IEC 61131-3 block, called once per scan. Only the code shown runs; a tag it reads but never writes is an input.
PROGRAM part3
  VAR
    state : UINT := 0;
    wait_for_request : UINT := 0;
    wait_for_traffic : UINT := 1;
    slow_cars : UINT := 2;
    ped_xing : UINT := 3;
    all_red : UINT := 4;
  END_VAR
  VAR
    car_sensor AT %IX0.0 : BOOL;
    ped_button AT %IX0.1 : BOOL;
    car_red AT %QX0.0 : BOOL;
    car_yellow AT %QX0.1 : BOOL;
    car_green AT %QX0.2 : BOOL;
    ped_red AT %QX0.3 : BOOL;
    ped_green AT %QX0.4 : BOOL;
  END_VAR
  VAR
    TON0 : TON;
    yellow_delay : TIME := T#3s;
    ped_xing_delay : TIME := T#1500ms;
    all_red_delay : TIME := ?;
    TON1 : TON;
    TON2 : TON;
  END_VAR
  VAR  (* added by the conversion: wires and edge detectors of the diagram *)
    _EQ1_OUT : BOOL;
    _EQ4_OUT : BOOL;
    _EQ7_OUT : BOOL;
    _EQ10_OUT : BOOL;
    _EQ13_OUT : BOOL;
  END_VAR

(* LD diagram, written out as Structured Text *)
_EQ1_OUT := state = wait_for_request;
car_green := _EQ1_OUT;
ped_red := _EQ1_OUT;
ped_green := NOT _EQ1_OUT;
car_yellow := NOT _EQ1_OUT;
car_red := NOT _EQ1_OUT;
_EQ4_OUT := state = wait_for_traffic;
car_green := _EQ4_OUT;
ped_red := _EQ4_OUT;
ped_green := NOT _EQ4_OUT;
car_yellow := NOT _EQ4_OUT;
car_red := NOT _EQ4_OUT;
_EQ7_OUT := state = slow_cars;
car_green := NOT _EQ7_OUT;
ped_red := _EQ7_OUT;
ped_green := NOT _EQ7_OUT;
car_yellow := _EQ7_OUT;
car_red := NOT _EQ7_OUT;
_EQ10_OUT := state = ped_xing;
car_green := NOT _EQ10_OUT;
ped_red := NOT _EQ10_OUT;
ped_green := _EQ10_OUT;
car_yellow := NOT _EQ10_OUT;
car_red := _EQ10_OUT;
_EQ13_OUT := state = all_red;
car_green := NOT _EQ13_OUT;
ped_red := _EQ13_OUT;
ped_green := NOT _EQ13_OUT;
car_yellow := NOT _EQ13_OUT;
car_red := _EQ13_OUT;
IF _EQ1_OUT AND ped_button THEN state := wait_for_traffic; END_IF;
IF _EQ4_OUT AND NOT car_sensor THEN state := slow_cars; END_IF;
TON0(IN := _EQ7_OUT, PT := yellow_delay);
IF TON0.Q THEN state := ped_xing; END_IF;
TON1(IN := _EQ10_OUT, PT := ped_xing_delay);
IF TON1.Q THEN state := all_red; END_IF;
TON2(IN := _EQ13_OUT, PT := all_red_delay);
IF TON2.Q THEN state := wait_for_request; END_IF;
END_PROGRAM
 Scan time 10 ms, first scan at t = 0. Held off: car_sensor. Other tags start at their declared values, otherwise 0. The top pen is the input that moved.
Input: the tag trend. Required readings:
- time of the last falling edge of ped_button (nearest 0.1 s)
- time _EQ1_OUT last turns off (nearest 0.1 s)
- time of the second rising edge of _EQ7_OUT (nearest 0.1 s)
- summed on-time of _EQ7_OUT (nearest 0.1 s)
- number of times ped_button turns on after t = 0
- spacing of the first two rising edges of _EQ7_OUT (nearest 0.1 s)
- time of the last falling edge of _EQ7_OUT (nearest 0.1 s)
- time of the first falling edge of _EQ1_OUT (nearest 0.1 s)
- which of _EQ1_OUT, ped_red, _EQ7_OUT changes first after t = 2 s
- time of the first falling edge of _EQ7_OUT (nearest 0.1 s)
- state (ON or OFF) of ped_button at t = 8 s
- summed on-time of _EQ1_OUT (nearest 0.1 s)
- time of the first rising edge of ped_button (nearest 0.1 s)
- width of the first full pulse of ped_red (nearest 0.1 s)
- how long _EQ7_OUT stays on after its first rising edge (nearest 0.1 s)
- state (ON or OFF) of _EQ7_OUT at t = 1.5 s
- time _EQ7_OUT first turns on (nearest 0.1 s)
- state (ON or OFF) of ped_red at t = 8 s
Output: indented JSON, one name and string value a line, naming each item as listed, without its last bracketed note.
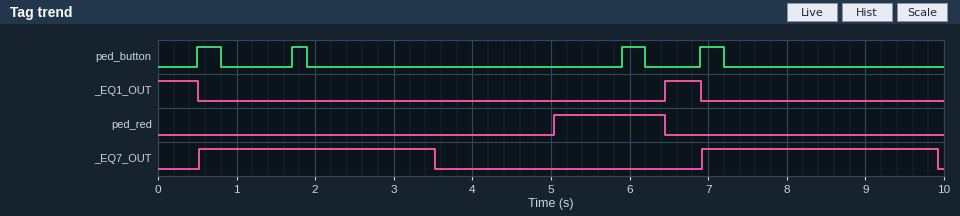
{
  "time of the last falling edge of ped_button": "7.2 s",
  "time _EQ1_OUT last turns off": "6.9 s",
  "time of the second rising edge of _EQ7_OUT": "6.9 s",
  "summed on-time of _EQ7_OUT": "6.0 s",
  "number of times ped_button turns on after t = 0": "4",
  "spacing of the first two rising edges of _EQ7_OUT": "6.4 s",
  "time of the last falling edge of _EQ7_OUT": "9.9 s",
  "time of the first falling edge of _EQ1_OUT": "0.5 s",
  "which of _EQ1_OUT, ped_red, _EQ7_OUT changes first after t = 2 s": "_EQ7_OUT",
  "time of the first falling edge of _EQ7_OUT": "3.5 s",
  "state (ON or OFF) of ped_button at t = 8 s": "OFF",
  "summed on-time of _EQ1_OUT": "1.0 s",
  "time of the first rising edge of ped_button": "0.5 s",
  "width of the first full pulse of ped_red": "1.4 s",
  "how long _EQ7_OUT stays on after its first rising edge": "3.0 s",
  "state (ON or OFF) of _EQ7_OUT at t = 1.5 s": "ON",
  "time _EQ7_OUT first turns on": "0.5 s",
  "state (ON or OFF) of ped_red at t = 8 s": "OFF"
}
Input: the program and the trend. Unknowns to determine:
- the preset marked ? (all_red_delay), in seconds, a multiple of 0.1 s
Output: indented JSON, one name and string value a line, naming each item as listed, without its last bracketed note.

{
  "the preset marked ? (all_red_delay), in seconds, a multiple of 0.1 s": "1.4 s"
}
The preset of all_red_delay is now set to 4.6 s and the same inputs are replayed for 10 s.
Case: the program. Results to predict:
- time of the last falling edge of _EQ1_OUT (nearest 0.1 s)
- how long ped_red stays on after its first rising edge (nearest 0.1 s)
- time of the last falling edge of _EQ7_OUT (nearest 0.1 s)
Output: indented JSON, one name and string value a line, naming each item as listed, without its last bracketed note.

{
  "time of the last falling edge of _EQ1_OUT": "0.5 s",
  "how long ped_red stays on after its first rising edge": "4.6 s",
  "time of the last falling edge of _EQ7_OUT": "3.5 s"
}
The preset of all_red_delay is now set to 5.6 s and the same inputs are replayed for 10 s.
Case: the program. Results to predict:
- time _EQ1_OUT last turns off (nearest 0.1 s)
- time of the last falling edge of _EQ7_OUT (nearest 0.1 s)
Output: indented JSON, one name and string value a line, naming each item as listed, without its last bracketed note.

{
  "time _EQ1_OUT last turns off": "0.5 s",
  "time of the last falling edge of _EQ7_OUT": "3.5 s"
}
